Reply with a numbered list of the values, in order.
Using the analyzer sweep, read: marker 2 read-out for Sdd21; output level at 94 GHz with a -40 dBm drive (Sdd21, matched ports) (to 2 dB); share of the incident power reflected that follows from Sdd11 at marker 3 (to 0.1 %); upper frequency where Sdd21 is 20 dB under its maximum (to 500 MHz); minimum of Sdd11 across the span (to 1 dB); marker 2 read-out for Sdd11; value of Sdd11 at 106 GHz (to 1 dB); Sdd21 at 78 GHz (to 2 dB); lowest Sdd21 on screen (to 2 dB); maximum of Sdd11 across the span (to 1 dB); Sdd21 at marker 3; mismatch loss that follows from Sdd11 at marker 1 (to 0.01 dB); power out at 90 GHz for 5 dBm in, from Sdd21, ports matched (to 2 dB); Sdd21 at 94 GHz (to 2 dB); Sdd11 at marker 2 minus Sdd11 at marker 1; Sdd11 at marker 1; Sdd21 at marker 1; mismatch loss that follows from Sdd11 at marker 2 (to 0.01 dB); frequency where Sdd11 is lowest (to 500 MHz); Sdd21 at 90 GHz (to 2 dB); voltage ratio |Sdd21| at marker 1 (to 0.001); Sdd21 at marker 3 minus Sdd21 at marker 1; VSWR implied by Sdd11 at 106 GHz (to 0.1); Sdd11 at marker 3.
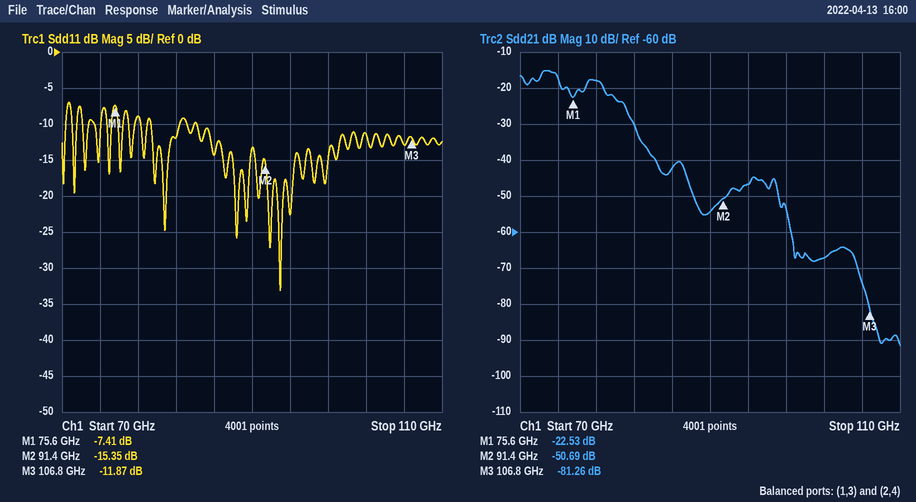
1. -50.69 dB
2. -86 dBm
3. 6.5 %
4. 83.0 GHz
5. -33 dB
6. -15.35 dB
7. -13 dB
8. -18 dB
9. -92 dB
10. -7 dB
11. -81.26 dB
12. 0.87 dB
13. -50 dBm
14. -46 dB
15. -7.94 dB
16. -7.41 dB
17. -22.53 dB
18. 0.13 dB
19. 93.0 GHz
20. -54 dB
21. 0.075
22. -58.73 dB
23. 1.6
24. -11.87 dB
